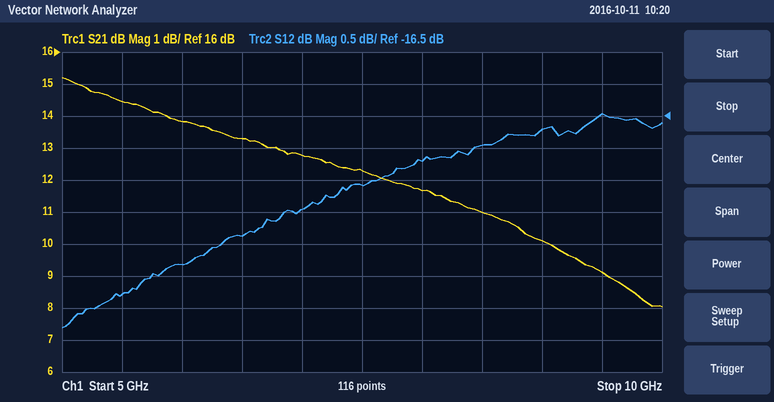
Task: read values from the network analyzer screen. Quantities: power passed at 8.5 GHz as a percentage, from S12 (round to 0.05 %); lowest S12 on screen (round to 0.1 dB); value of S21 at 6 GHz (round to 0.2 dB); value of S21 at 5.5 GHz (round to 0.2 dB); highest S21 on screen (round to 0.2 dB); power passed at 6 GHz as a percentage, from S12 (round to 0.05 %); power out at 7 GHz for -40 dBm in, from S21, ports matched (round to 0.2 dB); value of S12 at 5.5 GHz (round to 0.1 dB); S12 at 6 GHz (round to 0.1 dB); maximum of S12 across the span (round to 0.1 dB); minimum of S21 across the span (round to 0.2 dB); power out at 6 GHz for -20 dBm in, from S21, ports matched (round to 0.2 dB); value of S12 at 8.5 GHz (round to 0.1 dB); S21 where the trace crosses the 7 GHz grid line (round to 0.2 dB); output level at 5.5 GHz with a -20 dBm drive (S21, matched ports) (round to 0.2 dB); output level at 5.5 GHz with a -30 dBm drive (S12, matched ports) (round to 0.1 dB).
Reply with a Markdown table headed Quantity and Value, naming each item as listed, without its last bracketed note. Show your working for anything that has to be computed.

| Quantity | Value |
|---|---|
| power passed at 8.5 GHz as a percentage, from S12 | 10^(-17/10) ≈ 2.00 % |
| lowest S12 on screen | -19.8 dB |
| value of S21 at 6 GHz | 13.8 dB |
| value of S21 at 5.5 GHz | 14.4 dB |
| highest S21 on screen | 15.2 dB |
| power passed at 6 GHz as a percentage, from S12 | 10^(-18.8/10) ≈ 1.32 %, so 1.30 % to the nearest 0.05 % |
| power out at 7 GHz for -40 dBm in, from S21, ports matched | -40 dBm + (12.8 dB) = -27.2 dBm |
| value of S12 at 5.5 GHz | -19.3 dB |
| S12 at 6 GHz | -18.8 dB |
| maximum of S12 across the span | -16.5 dB |
| minimum of S21 across the span | 8.0 dB |
| power out at 6 GHz for -20 dBm in, from S21, ports matched | -20 dBm + (13.8 dB) = -6.2 dBm |
| value of S12 at 8.5 GHz | -17.0 dB |
| S21 where the trace crosses the 7 GHz grid line | 12.8 dB |
| output level at 5.5 GHz with a -20 dBm drive (S21, matched ports) | -20 dBm + (14.4 dB) = -5.6 dBm |
| output level at 5.5 GHz with a -30 dBm drive (S12, matched ports) | -30 dBm + (-19.3 dB) = -49.3 dBm |
